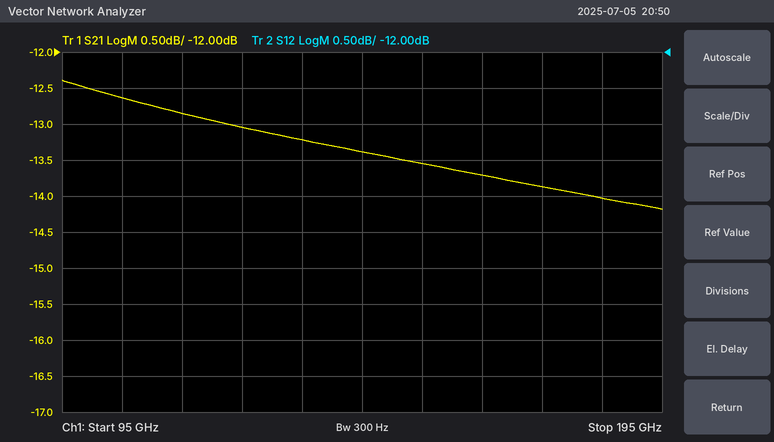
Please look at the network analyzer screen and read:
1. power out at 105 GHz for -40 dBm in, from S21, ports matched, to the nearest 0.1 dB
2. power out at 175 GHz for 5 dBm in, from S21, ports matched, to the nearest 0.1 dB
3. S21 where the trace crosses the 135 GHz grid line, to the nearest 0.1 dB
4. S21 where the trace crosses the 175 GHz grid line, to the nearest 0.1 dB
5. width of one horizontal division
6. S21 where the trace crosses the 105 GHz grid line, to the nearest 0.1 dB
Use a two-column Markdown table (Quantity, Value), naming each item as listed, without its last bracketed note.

| Quantity | Value |
|---|---|
| power out at 105 GHz for -40 dBm in, from S21, ports matched, to the nearest 0.1 dB | -52.6 dBm |
| power out at 175 GHz for 5 dBm in, from S21, ports matched, to the nearest 0.1 dB | -8.9 dBm |
| S21 where the trace crosses the 135 GHz grid line, to the nearest 0.1 dB | -13.2 dB |
| S21 where the trace crosses the 175 GHz grid line, to the nearest 0.1 dB | -13.9 dB |
| width of one horizontal division | 10 GHz |
| S21 where the trace crosses the 105 GHz grid line, to the nearest 0.1 dB | -12.6 dB |
